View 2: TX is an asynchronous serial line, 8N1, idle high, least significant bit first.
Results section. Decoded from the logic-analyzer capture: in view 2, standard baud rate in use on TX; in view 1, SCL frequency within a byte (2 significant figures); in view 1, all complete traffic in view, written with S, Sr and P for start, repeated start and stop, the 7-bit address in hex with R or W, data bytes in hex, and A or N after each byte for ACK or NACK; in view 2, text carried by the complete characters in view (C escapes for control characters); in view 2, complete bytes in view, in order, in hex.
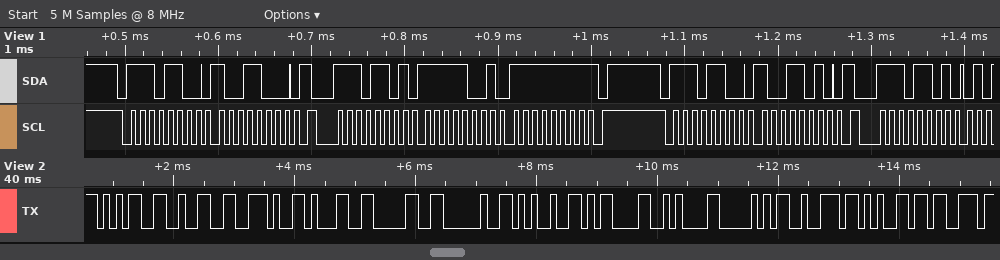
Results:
9600 baud
100 kHz
S 76W A 98 A Sr 76R A F9 A FF N P S 76W A 9A A Sr 76R A
"52.10 %\r\nPres"
35 32 2E 31 30 20 25 0D 0A 50 72 65 73
